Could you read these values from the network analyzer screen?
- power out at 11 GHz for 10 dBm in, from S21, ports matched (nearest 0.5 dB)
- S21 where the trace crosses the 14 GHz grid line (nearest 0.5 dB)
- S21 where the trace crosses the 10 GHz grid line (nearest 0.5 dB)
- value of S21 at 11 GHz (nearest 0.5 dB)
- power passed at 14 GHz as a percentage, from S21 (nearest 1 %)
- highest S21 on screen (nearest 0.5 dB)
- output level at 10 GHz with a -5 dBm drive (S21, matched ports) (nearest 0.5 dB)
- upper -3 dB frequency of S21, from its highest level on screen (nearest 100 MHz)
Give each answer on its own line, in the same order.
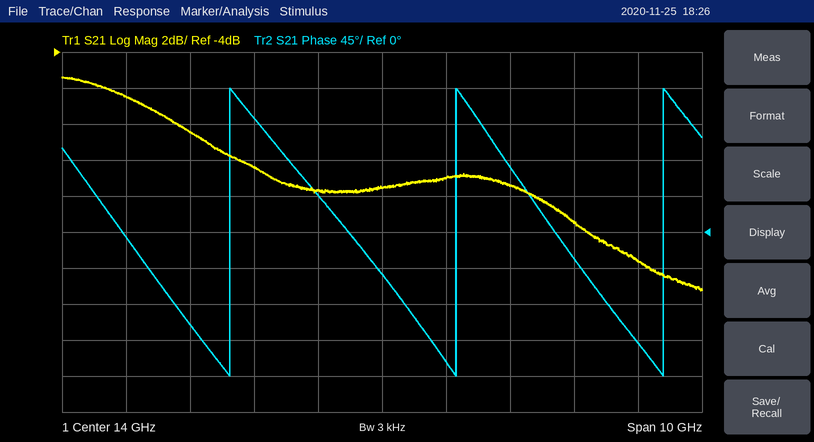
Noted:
1.5 dBm
-11.5 dB
-6.5 dB
-8.5 dB
7 %
-5.5 dB
-11.5 dBm
11.0 GHz
